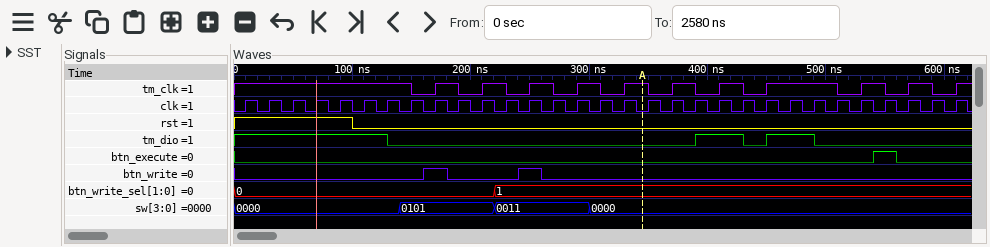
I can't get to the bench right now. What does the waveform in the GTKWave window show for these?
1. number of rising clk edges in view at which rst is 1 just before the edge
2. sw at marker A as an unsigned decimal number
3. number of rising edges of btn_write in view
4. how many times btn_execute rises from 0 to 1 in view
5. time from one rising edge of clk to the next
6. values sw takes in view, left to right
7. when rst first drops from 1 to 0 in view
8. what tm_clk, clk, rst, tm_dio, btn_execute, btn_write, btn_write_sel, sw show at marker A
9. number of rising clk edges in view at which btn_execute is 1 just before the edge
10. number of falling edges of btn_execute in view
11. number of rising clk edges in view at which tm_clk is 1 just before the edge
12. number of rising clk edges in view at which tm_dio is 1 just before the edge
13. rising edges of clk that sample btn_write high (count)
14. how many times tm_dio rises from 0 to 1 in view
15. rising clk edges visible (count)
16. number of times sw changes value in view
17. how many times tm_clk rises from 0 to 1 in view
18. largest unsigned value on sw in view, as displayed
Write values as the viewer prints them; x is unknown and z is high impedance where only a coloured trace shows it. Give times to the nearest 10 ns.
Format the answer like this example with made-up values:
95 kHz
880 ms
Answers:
5
0
2
1
20 ns
0000, 0101, 0011, 0000
100 ns
tm_clk=1, clk=0, rst=0, tm_dio=0, btn_execute=0, btn_write=0, btn_write_sel=1, sw=0000
1
1
20
11
2
2
31
3
11
0101
